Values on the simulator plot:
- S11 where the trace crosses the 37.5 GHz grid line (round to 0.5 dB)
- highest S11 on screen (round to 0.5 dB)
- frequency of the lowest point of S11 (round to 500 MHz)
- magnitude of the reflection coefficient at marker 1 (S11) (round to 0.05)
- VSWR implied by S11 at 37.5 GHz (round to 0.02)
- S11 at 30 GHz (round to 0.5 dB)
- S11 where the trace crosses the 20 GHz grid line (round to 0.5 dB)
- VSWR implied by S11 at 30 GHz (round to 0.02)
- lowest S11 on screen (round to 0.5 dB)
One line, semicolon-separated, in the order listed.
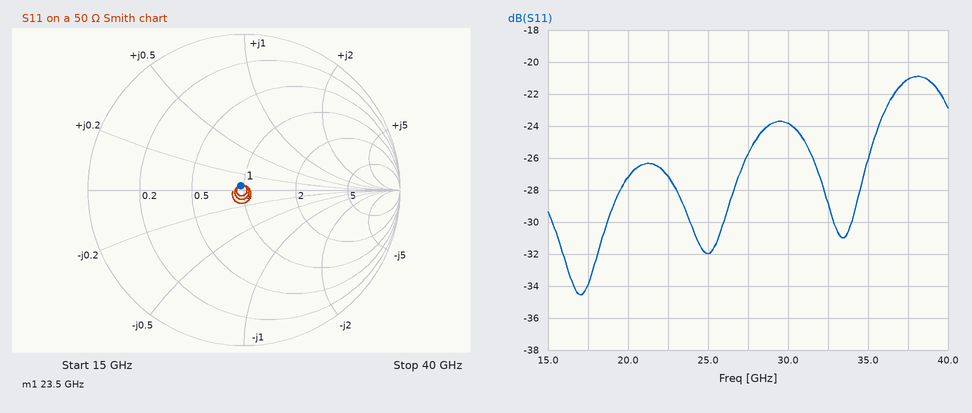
-21.0 dB; -21.0 dB; 17.0 GHz; 0.05; 1.20; -24.0 dB; -27.0 dB; 1.14; -34.5 dB
